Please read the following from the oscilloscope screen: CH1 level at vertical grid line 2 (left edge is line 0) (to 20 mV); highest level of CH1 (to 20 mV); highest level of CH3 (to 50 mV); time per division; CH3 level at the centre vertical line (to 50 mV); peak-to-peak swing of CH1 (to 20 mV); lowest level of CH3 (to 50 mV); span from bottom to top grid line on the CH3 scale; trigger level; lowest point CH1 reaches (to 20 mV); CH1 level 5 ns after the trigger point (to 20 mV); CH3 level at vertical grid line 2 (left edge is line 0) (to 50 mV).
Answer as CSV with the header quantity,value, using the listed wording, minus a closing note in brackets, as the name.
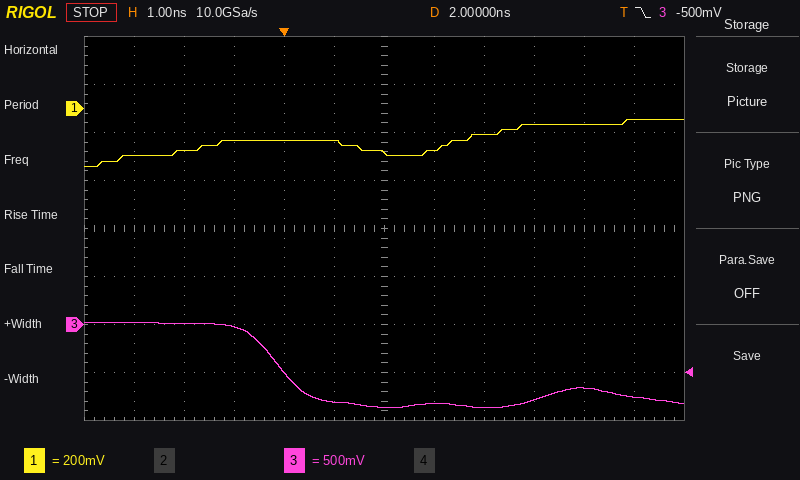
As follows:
quantity,value
CH1 level at vertical grid line 2 (left edge is line 0),-180 mV
highest level of CH1,-40 mV
highest level of CH3,0 mV
time per division,1 ns
CH3 level at the centre vertical line,-850 mV
peak-to-peak swing of CH1,200 mV
lowest level of CH3,-850 mV
span from bottom to top grid line on the CH3 scale,4 V
trigger level,-500 mV
lowest point CH1 reaches,-240 mV
CH1 level 5 ns after the trigger point,-60 mV
CH3 level at vertical grid line 2 (left edge is line 0),0 mV
